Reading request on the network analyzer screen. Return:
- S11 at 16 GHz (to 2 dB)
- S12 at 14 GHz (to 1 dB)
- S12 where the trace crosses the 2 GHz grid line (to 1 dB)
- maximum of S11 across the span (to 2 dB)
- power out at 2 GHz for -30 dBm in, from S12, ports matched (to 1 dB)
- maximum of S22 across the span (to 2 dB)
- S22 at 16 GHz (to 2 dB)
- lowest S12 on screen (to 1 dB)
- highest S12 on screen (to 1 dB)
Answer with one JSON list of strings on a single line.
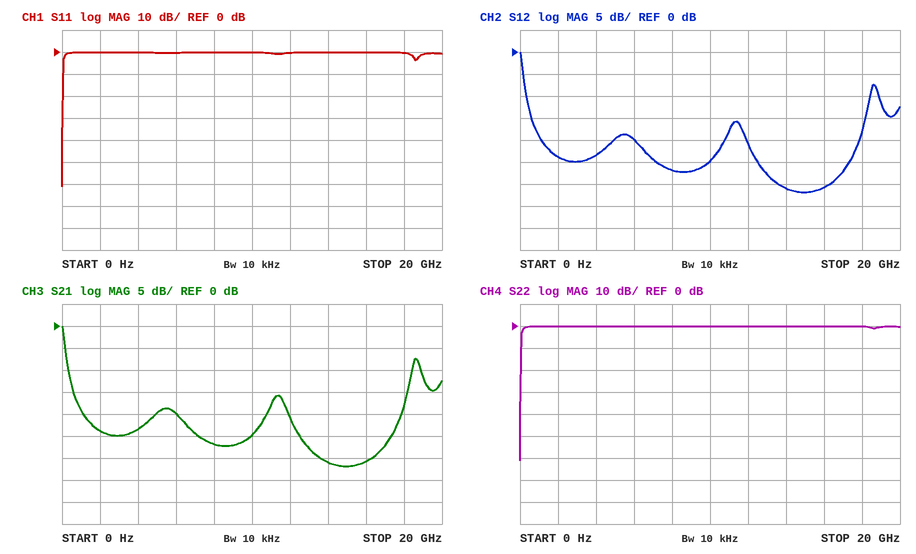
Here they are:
["0 dB", "-31 dB", "-24 dB", "0 dB", "-54 dBm", "0 dB", "0 dB", "-32 dB", "0 dB"]
